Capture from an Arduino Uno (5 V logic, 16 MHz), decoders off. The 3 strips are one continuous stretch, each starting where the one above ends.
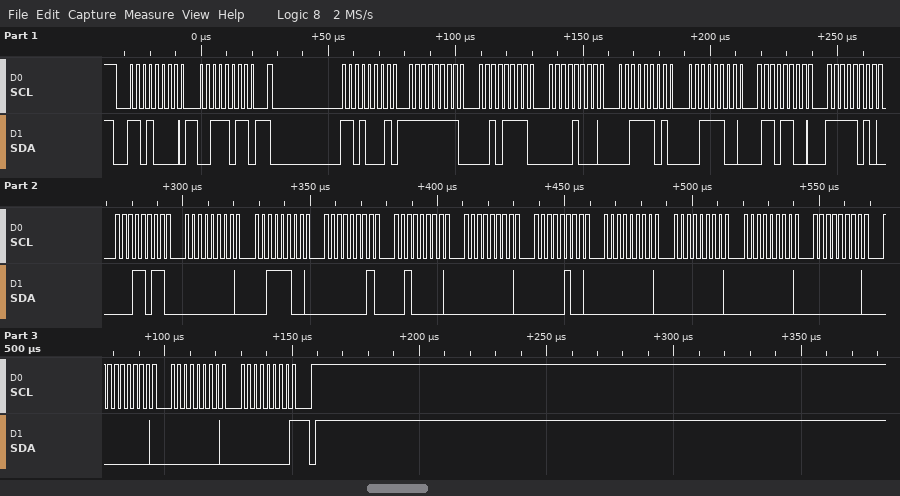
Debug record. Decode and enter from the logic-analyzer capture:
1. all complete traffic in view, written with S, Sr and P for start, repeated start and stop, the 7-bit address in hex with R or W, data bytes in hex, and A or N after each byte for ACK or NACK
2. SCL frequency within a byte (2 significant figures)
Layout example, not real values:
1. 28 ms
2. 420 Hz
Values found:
1. S 68W A 3B A Sr 68R A FF A 2F A 08 A 3D A 3C A 6C A FA A 1B A 00 A 3C A 01 A 20 A 00 A 04 A 00 A 00 A 00 A 00 A 00 A 00 A 00 N P
2. 400 kHz
